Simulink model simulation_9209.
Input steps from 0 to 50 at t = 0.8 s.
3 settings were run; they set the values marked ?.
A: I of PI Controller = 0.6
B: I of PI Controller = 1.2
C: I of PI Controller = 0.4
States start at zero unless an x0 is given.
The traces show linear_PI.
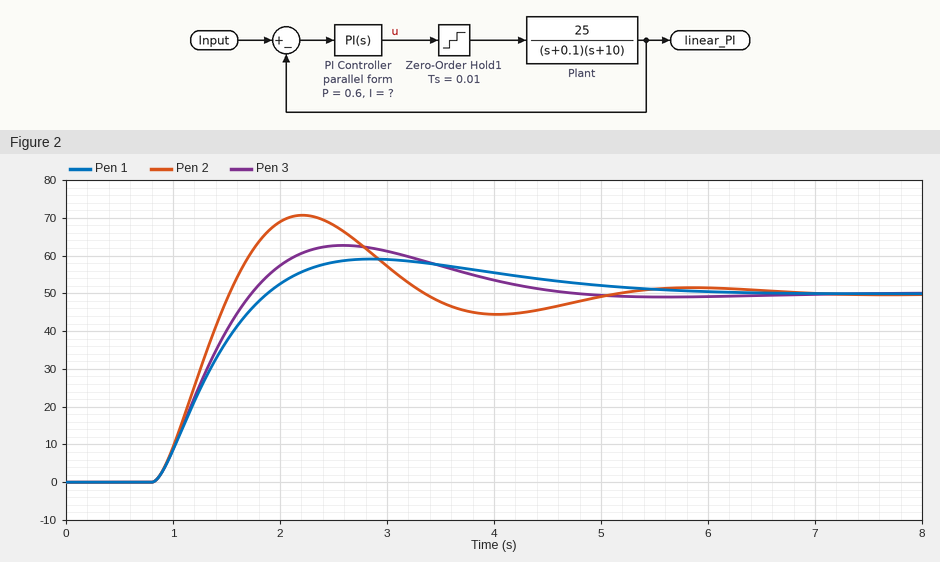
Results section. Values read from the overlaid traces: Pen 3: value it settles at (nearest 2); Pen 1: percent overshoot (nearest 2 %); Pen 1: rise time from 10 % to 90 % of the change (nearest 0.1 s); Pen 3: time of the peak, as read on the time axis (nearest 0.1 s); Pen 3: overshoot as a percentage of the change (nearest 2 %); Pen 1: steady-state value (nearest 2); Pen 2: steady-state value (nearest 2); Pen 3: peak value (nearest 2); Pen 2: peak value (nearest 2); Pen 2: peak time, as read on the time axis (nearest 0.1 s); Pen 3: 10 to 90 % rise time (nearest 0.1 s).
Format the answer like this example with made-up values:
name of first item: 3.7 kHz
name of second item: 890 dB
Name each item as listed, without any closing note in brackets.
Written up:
Pen 3: value it settles at: 50
Pen 1: percent overshoot: 18 %
Pen 1: rise time from 10 % to 90 % of the change: 0.8 s
Pen 3: time of the peak, as read on the time axis: 2.6 s
Pen 3: overshoot as a percentage of the change: 26 %
Pen 1: steady-state value: 50
Pen 2: steady-state value: 50
Pen 3: peak value: 62
Pen 2: peak value: 70
Pen 2: peak time, as read on the time axis: 2.2 s
Pen 3: 10 to 90 % rise time: 0.7 s
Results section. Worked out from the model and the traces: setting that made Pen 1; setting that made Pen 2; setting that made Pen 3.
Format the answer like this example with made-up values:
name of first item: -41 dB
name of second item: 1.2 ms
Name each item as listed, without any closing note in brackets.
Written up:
setting that made Pen 1: C
setting that made Pen 2: B
setting that made Pen 3: A
